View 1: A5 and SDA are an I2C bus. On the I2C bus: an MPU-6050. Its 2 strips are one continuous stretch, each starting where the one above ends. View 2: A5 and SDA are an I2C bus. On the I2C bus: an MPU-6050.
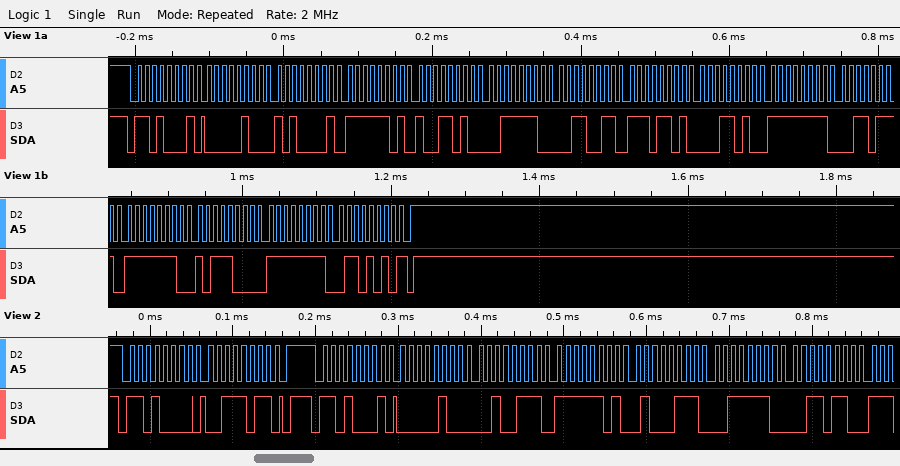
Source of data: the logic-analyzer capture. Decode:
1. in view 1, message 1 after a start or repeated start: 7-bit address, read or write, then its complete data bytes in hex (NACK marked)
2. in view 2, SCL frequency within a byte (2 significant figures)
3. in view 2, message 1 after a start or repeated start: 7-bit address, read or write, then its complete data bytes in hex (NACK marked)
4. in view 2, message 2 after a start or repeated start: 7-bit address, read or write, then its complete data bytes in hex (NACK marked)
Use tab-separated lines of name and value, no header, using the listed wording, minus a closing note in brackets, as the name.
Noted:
in view 1, message 1 after a start or repeated start: 7-bit address, read or write, then its complete data bytes in hex	0x68 read: 04 A1 FD 9A 3E 33 ED 1A FF 37 FE B8 FF 6A NACK
in view 2, SCL frequency within a byte	100 kHz
in view 2, message 1 after a start or repeated start: 7-bit address, read or write, then its complete data bytes in hex	0x68 write: 3B
in view 2, message 2 after a start or repeated start: 7-bit address, read or write, then its complete data bytes in hex	0x68 read: 04 27 FD 47 3E 36
